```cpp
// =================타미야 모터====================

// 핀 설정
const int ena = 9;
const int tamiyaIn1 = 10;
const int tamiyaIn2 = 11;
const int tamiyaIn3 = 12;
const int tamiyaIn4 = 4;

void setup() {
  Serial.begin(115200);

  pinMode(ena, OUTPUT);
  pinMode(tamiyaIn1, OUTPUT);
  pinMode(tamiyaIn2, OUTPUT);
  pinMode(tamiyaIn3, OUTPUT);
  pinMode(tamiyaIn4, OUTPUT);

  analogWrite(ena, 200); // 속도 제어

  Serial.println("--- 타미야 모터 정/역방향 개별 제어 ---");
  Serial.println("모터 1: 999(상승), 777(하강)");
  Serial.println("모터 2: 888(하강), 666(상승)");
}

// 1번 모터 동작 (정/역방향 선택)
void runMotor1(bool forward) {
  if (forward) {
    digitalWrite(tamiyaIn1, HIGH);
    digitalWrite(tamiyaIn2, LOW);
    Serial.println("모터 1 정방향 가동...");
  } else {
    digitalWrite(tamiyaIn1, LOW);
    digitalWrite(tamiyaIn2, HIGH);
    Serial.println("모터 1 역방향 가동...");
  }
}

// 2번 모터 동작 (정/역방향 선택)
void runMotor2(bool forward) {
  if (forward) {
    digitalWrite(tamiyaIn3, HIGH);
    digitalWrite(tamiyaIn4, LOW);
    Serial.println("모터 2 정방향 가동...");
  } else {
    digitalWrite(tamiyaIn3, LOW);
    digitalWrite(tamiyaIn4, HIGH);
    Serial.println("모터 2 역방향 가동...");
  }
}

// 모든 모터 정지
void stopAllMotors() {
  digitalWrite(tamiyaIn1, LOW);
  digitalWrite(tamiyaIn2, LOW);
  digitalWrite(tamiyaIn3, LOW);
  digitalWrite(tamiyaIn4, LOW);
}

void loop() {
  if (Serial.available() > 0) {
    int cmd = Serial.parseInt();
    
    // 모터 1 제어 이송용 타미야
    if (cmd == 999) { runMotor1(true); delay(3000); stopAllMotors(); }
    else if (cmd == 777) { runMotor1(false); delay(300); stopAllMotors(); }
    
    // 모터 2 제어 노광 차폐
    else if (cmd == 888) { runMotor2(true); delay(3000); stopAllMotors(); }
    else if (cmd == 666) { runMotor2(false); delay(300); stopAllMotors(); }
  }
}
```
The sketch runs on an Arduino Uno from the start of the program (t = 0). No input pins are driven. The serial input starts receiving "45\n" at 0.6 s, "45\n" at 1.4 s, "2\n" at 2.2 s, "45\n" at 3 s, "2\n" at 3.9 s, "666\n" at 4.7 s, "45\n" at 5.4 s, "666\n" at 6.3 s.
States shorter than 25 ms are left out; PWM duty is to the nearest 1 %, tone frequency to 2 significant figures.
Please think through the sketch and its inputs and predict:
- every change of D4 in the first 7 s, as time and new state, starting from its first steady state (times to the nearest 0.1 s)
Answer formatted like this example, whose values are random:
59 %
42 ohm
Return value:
0 s low; 4.7 s high; 5 s low; 6.3 s high; 6.6 s low
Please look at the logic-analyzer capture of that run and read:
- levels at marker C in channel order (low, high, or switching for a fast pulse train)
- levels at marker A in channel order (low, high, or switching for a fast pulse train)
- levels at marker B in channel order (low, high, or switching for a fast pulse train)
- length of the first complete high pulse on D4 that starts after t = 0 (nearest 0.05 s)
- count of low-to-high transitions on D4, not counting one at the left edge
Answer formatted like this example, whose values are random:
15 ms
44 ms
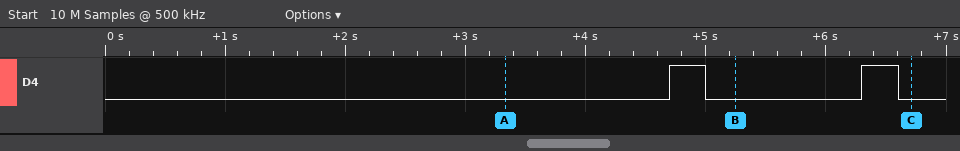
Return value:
D4 low
D4 low
D4 low
0.30 s
2
